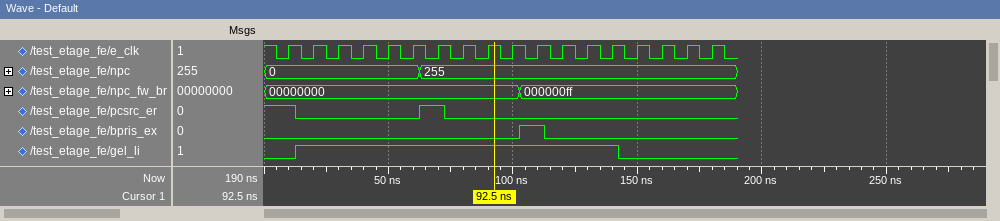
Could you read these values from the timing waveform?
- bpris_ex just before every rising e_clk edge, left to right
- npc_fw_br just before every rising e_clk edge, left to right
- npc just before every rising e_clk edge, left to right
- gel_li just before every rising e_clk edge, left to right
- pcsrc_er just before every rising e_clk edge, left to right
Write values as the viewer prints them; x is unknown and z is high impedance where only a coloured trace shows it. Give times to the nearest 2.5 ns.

0 0 0 0 0 0 0 0 0 0 1 0 0 0 0 0 0 0
00000000, 00000000, 00000000, 00000000, 00000000, 00000000, 00000000, 00000000, 00000000, 00000000, 000000ff, 000000ff, 000000ff, 000000ff, 000000ff, 000000ff, 000000ff, 000000ff
0, 0, 0, 0, 0, 0, 255, 255, 255, 255, 255, 255, 255, 255, 255, 255, 255, 255
0 1 1 1 1 1 1 1 1 1 1 1 1 1 0 0 0 0
1 0 0 0 0 0 1 0 0 0 0 0 0 0 0 0 0 0
